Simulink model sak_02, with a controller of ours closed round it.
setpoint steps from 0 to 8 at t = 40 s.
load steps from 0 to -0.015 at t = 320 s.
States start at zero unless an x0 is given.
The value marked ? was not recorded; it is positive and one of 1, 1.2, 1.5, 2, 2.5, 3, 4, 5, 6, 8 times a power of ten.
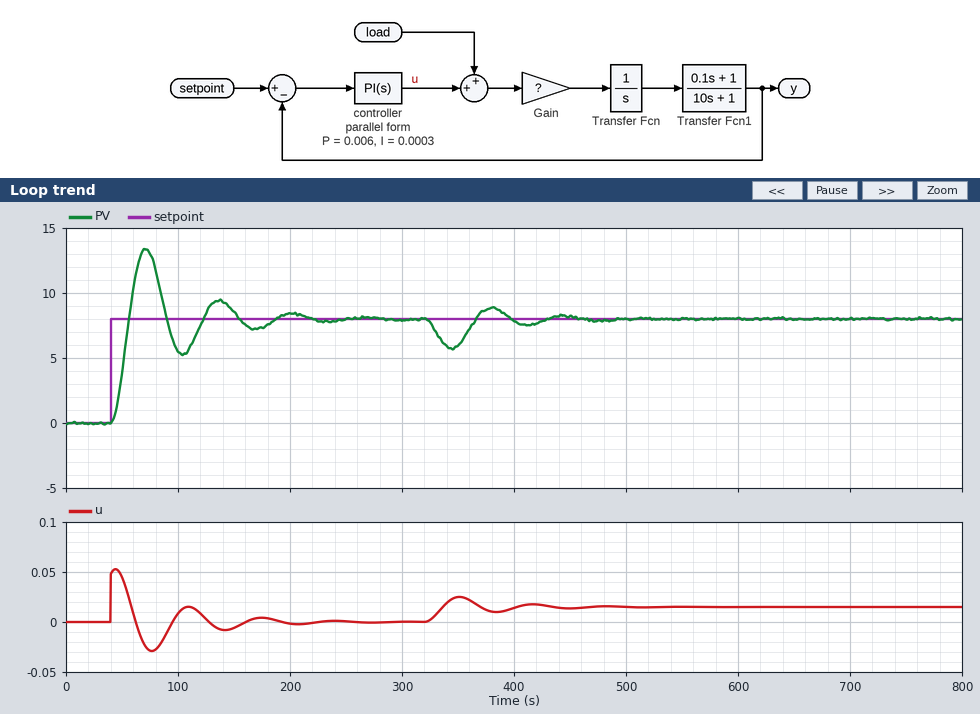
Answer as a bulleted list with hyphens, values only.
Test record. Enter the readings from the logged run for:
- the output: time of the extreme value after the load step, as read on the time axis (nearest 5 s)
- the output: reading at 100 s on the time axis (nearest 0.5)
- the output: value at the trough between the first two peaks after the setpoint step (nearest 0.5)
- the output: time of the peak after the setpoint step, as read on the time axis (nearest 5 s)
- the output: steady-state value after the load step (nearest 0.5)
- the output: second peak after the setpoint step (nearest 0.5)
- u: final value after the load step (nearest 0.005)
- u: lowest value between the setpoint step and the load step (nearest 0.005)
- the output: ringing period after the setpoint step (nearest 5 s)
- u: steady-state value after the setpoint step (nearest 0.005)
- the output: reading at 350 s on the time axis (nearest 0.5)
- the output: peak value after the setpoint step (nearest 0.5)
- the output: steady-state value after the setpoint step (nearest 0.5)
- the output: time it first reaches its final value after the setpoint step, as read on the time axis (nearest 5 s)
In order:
- 345 s
- 5.5
- 5.5
- 70 s
- 8.0
- 9.5
- 0.015
- -0.030
- 65 s
- 0.000
- 6.0
- 13.5
- 8.0
- 55 s
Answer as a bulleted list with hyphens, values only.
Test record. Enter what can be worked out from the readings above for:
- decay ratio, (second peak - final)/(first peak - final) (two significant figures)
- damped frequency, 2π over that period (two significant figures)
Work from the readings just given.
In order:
- 0.27
- 0.097 rad/s
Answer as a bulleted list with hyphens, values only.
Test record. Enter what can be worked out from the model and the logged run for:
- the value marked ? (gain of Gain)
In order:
- 20
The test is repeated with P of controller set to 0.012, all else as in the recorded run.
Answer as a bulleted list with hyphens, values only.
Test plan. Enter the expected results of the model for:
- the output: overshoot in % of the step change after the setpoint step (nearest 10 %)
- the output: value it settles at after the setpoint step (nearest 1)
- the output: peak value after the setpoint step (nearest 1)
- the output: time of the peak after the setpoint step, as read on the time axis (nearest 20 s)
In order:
- 50 %
- 8
- 12
- 60 s
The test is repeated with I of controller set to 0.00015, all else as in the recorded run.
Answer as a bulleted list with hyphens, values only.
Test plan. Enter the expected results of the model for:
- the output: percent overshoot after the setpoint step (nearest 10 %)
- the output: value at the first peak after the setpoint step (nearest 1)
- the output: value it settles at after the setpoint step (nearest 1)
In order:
- 50 %
- 12
- 8
